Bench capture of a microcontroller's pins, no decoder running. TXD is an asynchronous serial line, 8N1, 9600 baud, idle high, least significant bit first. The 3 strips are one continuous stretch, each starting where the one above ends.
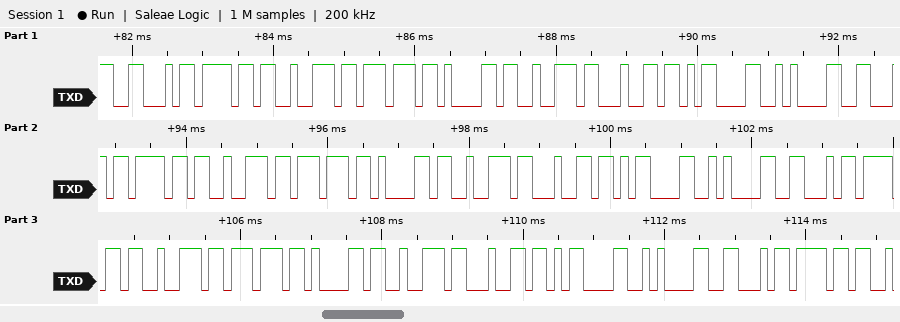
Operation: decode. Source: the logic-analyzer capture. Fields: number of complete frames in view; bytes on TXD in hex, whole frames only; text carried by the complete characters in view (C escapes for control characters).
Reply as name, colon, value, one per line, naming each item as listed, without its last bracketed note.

number of complete frames in view: 29
bytes on TXD in hex, whole frames only: 46 6F 72 77 61 72 64 0D 0A 46 6F 72 77 61 72 64 0D 0A 46 6F 72 77 61 72 64 0D 0A 46 6F
text carried by the complete characters in view: "Forward\r\nForward\r\nForward\r\nFo"
